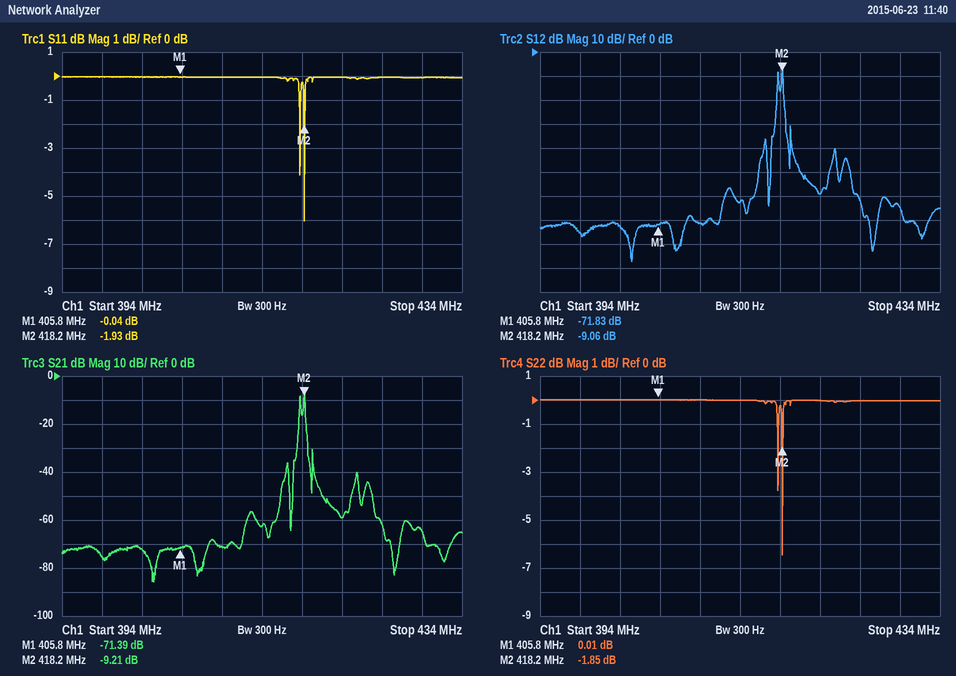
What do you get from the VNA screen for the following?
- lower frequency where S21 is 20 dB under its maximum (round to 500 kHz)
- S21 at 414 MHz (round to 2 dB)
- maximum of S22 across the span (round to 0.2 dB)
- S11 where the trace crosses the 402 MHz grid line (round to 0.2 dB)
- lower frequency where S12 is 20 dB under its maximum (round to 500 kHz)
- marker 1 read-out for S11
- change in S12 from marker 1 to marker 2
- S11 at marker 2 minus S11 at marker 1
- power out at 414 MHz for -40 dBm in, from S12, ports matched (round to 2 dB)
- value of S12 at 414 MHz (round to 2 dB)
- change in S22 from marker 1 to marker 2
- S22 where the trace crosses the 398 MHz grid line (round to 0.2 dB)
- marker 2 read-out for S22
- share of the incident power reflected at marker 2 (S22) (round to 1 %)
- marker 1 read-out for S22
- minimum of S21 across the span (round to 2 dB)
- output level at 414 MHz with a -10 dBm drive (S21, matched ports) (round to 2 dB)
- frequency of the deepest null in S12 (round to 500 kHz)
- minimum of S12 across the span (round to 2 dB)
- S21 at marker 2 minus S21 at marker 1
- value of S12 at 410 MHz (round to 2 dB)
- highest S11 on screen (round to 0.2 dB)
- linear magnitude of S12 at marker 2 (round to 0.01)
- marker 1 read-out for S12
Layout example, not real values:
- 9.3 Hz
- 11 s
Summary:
- 417.5 MHz
- -62 dB
- 0.0 dB
- 0.0 dB
- 417.5 MHz
- -0.04 dB
- 62.77 dB
- -1.89 dB
- -102 dBm
- -62 dB
- -1.86 dB
- 0.0 dB
- -1.85 dB
- 65 %
- 0.01 dB
- -86 dB
- -72 dBm
- 403.0 MHz
- -88 dB
- 62.18 dB
- -72 dB
- 0.0 dB
- 0.35
- -71.83 dB
